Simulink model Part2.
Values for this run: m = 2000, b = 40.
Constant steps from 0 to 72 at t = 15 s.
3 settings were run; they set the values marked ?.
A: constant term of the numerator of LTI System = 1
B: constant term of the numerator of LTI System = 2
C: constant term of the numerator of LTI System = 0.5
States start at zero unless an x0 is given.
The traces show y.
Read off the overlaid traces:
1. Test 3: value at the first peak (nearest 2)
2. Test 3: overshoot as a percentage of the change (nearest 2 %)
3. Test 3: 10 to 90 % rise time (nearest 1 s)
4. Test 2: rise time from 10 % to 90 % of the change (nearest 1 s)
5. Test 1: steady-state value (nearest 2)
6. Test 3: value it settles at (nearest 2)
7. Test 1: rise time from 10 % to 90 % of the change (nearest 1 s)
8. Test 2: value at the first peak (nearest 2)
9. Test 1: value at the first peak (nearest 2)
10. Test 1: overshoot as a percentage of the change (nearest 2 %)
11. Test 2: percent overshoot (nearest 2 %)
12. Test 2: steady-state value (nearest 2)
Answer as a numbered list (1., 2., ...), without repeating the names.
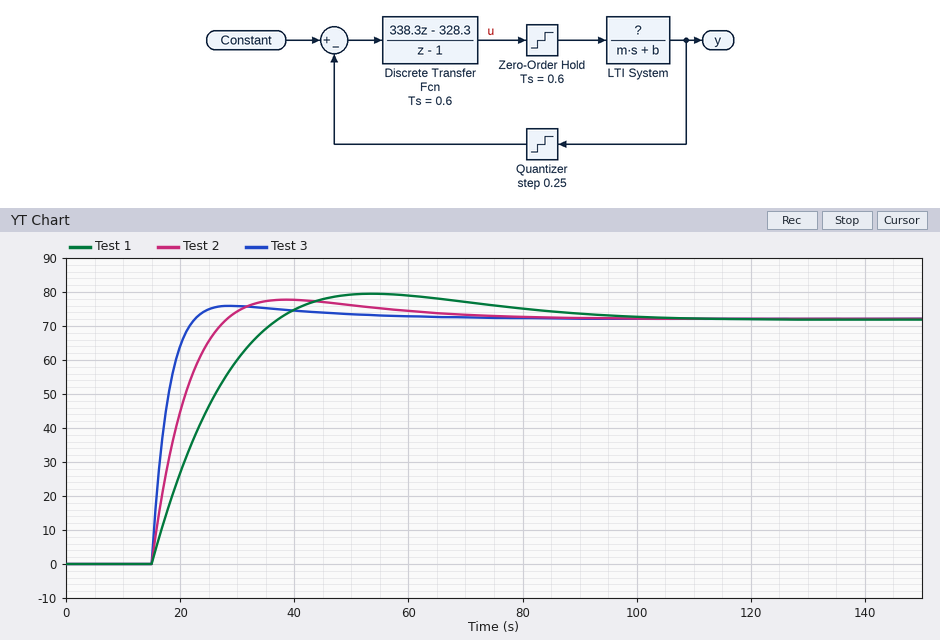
1. 76
2. 6 %
3. 5 s
4. 9 s
5. 72
6. 72
7. 16 s
8. 78
9. 80
10. 10 %
11. 8 %
12. 72
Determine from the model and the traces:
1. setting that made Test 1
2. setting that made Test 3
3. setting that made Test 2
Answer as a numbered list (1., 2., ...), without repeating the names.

1. C
2. B
3. A
